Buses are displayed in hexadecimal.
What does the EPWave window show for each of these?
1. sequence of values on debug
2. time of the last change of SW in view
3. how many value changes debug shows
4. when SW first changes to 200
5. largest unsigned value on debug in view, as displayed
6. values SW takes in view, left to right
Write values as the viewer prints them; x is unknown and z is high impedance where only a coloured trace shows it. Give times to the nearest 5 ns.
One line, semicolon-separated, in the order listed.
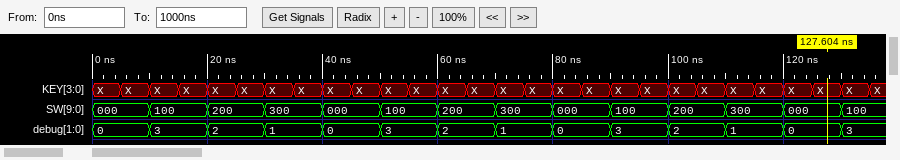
0, 3, 2, 1, 0, 3, 2, 1, 0, 3, 2, 1, 0, 3; 130 ns; 13; 20 ns; 3; 000, 100, 200, 300, 000, 100, 200, 300, 000, 100, 200, 300, 000, 100
